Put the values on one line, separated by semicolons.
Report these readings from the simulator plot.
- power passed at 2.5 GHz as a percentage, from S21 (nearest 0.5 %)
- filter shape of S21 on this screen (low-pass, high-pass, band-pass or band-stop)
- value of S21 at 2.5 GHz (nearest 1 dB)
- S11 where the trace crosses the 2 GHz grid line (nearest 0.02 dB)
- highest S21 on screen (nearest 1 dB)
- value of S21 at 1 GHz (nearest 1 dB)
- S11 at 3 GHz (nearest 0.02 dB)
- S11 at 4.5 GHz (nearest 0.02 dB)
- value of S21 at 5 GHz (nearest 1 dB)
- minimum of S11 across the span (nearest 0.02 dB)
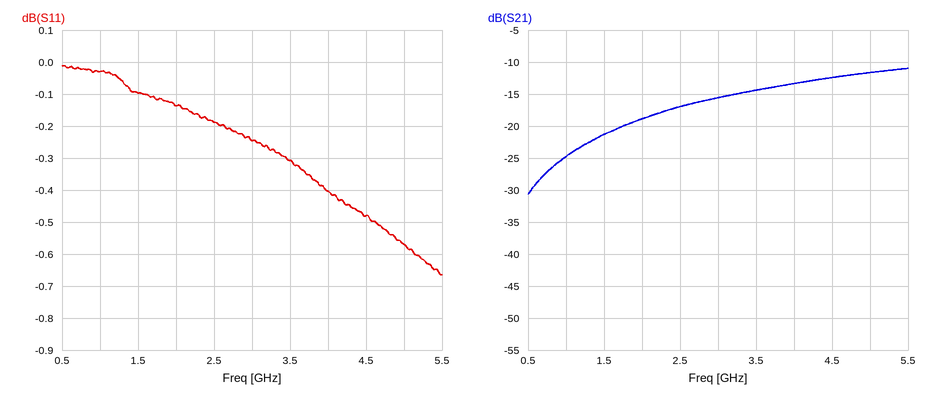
2.0 %; high-pass; -17 dB; -0.14 dB; -11 dB; -25 dB; -0.24 dB; -0.48 dB; -12 dB; -0.66 dB
